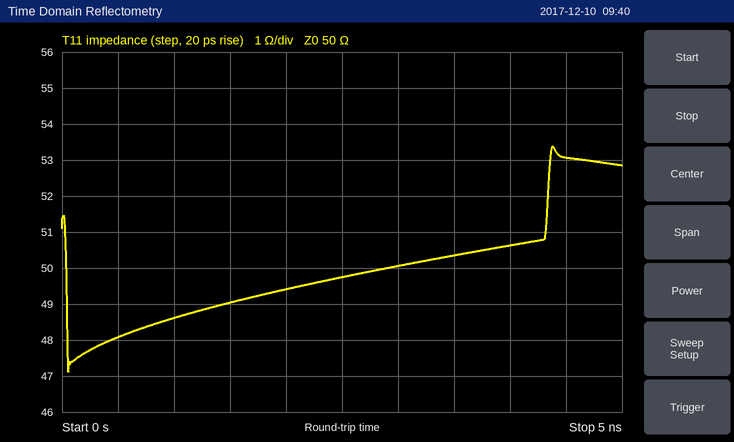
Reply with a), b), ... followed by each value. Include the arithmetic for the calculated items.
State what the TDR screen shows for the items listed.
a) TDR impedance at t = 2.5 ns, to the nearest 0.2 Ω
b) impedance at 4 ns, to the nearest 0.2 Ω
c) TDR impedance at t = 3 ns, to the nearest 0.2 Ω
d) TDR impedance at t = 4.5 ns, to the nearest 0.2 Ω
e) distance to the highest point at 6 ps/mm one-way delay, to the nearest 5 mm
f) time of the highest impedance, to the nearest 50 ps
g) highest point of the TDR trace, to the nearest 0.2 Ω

a) 49.8 Ω
b) 50.6 Ω
c) 50.0 Ω
d) 53.0 Ω
e) 4.40 ns / 2 / 6 ps/mm ≈ 367 mm, so 365 mm to the nearest 5 mm
f) 4.40 ns
g) 53.4 Ω
